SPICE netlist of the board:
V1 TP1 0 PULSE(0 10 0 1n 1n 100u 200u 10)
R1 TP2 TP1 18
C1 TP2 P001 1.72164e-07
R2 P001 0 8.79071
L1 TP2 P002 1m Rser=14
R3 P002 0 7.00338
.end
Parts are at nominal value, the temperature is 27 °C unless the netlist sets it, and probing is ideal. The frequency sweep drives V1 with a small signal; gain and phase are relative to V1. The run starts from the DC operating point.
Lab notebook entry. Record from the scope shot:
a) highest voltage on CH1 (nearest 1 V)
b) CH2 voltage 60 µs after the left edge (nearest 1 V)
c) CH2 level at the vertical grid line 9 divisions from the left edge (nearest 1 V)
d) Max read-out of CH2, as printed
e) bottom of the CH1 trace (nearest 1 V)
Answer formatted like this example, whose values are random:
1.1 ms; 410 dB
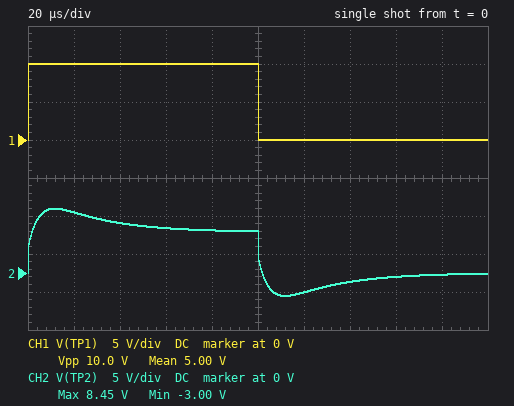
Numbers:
10 V; 6 V; 0 V; 8.45 V; 0 V
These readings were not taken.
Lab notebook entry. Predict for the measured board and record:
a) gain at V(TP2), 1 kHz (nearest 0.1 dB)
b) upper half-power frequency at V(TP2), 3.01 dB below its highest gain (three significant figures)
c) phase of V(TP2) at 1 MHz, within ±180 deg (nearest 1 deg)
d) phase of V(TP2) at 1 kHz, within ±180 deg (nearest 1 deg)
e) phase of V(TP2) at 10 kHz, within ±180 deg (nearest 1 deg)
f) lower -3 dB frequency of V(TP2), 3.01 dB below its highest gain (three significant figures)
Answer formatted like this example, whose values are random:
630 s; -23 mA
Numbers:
-5.1 dB; 48.0 kHz; -4 deg; 7 deg; 3 deg; 2.91 kHz
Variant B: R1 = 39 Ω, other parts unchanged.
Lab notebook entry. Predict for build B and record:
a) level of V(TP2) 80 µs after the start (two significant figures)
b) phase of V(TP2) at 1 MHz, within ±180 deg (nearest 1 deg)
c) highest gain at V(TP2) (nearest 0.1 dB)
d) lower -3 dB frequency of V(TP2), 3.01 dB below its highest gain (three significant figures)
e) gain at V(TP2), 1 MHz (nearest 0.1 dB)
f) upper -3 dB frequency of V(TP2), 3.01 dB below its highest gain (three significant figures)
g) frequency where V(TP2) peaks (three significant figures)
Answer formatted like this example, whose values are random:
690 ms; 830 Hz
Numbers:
3.5 V; -5 deg; -1.5 dB; 5.19 kHz; -14.7 dB; 30.3 kHz; 13.1 kHz
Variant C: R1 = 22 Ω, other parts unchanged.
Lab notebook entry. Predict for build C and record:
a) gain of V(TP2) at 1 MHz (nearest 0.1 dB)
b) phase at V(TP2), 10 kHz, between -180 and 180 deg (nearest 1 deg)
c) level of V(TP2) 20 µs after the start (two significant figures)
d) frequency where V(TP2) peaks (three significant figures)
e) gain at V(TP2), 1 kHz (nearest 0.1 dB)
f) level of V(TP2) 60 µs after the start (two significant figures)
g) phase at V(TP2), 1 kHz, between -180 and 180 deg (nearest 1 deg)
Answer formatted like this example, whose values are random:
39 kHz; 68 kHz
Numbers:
-10.8 dB; 4 deg; 7.7 V; 13.5 kHz; -5.9 dB; 5.3 V; 8 deg
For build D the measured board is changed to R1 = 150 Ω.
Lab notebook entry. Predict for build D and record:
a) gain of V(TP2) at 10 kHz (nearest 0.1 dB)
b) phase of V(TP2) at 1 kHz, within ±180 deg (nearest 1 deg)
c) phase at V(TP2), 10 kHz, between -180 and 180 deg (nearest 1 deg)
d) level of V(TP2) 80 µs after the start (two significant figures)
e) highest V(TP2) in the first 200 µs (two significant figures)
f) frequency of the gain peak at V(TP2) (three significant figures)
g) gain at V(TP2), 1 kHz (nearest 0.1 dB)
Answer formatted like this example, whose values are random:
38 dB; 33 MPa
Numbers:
-5.8 dB; 13 deg; 16 deg; 1.0 V; 3.5 V; 12.5 kHz; -17.8 dB
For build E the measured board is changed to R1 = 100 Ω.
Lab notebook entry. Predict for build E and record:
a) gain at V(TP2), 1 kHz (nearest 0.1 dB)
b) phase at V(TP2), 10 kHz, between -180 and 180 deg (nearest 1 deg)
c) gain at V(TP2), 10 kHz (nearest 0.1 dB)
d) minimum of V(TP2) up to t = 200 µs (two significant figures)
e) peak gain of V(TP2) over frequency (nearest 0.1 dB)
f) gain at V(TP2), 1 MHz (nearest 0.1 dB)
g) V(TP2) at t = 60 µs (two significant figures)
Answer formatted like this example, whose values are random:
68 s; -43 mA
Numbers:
-14.8 dB; 13 deg; -4.2 dB; -2.7 V; -3.4 dB; -21.8 dB; 1.3 V
